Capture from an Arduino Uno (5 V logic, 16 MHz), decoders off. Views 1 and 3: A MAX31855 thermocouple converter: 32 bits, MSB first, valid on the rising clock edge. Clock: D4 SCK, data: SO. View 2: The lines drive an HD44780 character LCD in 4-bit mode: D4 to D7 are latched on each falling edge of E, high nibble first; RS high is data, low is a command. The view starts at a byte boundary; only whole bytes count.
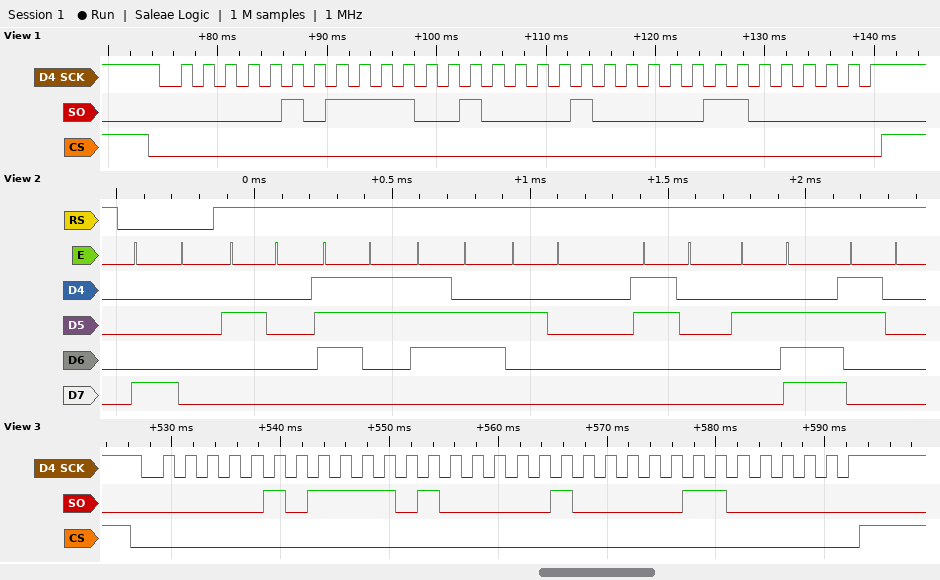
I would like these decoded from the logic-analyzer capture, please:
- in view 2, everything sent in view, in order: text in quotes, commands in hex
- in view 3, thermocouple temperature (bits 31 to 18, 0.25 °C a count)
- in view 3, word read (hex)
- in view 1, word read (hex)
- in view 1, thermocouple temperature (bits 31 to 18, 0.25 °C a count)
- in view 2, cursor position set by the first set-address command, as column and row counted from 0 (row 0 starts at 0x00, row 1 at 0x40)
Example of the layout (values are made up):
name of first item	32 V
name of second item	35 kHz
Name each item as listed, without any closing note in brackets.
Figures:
in view 2, everything sent in view, in order: text in quotes, commands in hex	0x80 " sv 0.0"
in view 3, thermocouple temperature	94.50 °C
in view 3, word read	0x05E820C0
in view 1, word read	0x05E420C0
in view 1, thermocouple temperature	94.25 °C
in view 2, cursor position set by the first set-address command, as column and row counted from 0	column 0, row 0
